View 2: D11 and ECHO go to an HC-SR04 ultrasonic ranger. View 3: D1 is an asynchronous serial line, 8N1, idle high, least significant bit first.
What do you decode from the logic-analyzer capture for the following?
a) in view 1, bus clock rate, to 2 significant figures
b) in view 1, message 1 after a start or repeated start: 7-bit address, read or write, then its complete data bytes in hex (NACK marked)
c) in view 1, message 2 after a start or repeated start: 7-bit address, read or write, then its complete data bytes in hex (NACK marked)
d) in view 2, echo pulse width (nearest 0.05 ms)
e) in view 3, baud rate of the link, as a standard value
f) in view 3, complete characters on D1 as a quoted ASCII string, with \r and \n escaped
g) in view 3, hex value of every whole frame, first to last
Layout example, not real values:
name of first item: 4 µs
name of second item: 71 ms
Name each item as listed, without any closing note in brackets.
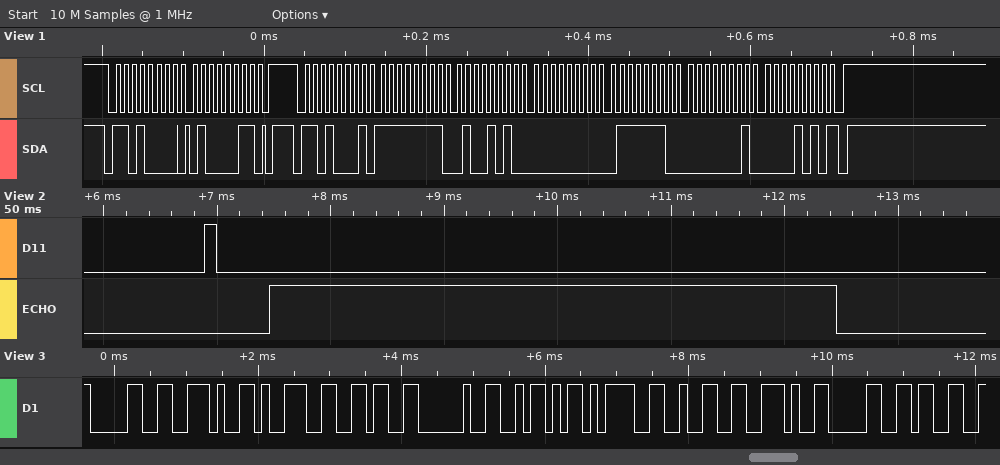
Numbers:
in view 1, bus clock rate, to 2 significant figures: 100 kHz
in view 1, message 1 after a start or repeated start: 7-bit address, read or write, then its complete data bytes in hex: 0x68 write: 43
in view 1, message 2 after a start or repeated start: 7-bit address, read or write, then its complete data bytes in hex: 0x68 read: FF 4A 00 7E 01 0A NACK
in view 2, echo pulse width: 5.00 ms
in view 3, baud rate of the link, as a standard value: 9600 baud
in view 3, complete characters on D1 as a quoted ASCII string, with \r and \n escaped: "0.96 Z=2.03"
in view 3, hex value of every whole frame, first to last: 30 2E 39 36 20 5A 3D 32 2E 30 33
